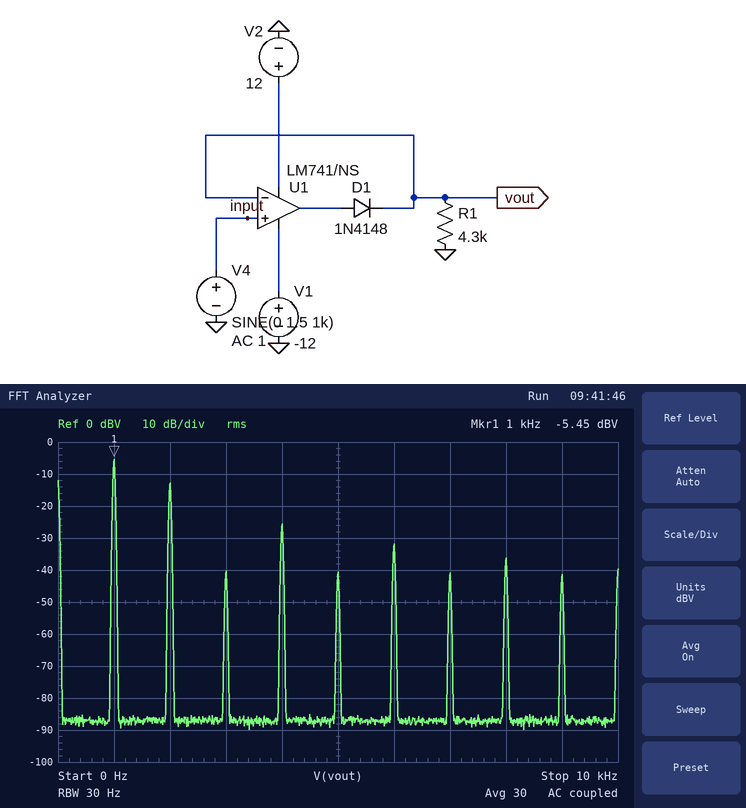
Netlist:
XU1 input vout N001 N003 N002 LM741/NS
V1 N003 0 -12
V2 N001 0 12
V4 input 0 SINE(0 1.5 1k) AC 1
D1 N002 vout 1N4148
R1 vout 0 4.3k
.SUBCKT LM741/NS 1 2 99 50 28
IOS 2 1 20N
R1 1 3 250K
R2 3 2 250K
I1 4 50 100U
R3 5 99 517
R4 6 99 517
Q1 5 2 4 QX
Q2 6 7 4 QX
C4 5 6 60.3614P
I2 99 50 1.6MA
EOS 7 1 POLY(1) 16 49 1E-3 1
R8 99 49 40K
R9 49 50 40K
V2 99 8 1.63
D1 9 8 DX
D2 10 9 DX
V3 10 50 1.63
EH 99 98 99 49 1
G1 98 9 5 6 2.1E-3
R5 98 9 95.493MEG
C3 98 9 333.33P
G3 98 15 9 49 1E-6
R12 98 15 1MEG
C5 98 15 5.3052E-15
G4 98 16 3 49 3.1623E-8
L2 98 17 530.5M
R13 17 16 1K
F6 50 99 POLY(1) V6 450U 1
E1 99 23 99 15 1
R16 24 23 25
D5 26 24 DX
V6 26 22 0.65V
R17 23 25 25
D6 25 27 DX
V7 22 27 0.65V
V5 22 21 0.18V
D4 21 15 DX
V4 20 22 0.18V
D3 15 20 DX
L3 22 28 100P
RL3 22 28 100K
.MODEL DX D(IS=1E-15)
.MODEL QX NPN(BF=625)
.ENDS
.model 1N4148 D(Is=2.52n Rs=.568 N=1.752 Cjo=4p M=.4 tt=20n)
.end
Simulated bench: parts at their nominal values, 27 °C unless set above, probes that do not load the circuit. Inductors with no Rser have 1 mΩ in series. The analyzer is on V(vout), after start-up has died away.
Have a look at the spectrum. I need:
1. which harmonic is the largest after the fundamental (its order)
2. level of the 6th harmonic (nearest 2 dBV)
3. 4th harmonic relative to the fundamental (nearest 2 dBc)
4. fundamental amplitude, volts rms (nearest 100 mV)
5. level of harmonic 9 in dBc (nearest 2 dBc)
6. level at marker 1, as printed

2
-32 dBV
-20 dBc
500 mV
-36 dBc
-5.45 dBV
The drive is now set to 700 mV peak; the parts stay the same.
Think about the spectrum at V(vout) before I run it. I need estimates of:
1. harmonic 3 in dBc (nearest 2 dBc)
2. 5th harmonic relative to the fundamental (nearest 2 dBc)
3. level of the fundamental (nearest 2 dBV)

-34 dBc
-34 dBc
-12 dBV
